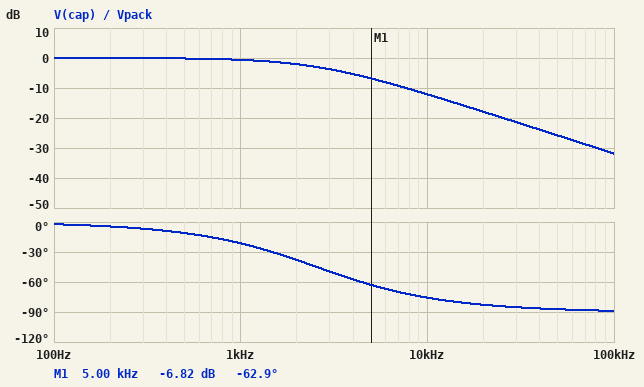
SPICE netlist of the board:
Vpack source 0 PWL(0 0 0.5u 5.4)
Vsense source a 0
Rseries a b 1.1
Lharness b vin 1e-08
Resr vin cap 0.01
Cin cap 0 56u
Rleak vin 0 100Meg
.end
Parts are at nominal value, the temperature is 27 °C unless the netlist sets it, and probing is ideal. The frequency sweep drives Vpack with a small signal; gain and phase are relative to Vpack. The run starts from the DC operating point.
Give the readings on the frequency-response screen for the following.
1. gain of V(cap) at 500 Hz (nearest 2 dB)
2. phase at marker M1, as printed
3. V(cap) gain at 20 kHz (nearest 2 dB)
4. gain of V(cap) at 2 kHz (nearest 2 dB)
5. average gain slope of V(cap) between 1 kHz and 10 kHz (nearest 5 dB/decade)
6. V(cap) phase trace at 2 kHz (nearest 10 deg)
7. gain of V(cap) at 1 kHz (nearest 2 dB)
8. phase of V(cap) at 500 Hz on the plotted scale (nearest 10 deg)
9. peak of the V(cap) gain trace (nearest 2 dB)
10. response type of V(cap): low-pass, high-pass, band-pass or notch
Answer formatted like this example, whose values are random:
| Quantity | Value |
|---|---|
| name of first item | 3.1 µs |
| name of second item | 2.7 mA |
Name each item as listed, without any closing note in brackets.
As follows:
| Quantity | Value |
|---|---|
| gain of V(cap) at 500 Hz | 0 dB |
| phase at marker M1, as printed | -62.9 deg |
| V(cap) gain at 20 kHz | -18 dB |
| gain of V(cap) at 2 kHz | -2 dB |
| average gain slope of V(cap) between 1 kHz and 10 kHz | -10 dB/decade |
| V(cap) phase trace at 2 kHz | -40 deg |
| gain of V(cap) at 1 kHz | 0 dB |
| phase of V(cap) at 500 Hz on the plotted scale | -10 deg |
| peak of the V(cap) gain trace | 0 dB |
| response type of V(cap): low-pass, high-pass, band-pass or notch | low-pass |
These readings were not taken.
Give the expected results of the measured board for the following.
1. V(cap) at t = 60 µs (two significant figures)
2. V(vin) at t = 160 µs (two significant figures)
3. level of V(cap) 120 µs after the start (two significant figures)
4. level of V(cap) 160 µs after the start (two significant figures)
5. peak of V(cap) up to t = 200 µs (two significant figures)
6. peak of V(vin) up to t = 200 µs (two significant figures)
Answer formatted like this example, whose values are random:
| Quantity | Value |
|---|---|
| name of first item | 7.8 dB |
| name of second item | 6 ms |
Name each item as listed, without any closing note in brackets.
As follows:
| Quantity | Value |
|---|---|
| V(cap) at t = 60 µs | 3.3 V |
| V(vin) at t = 160 µs | 5.0 V |
| level of V(cap) 120 µs after the start | 4.6 V |
| level of V(cap) 160 µs after the start | 5.0 V |
| peak of V(cap) up to t = 200 µs | 5.2 V |
| peak of V(vin) up to t = 200 µs | 5.2 V |
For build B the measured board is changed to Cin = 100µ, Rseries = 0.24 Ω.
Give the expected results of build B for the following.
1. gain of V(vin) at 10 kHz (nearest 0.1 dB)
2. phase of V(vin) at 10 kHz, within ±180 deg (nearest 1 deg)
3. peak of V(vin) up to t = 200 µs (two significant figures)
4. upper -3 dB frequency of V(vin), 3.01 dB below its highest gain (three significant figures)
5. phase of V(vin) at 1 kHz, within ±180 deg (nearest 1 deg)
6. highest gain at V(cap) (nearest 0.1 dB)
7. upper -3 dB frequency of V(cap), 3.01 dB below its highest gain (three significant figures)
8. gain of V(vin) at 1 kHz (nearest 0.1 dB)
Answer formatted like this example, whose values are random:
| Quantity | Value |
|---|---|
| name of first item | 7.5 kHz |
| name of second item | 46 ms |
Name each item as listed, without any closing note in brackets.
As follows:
| Quantity | Value |
|---|---|
| gain of V(vin) at 10 kHz | -5.4 dB |
| phase of V(vin) at 10 kHz, within ±180 deg | -54 deg |
| peak of V(vin) up to t = 200 µs | 5.4 V |
| upper -3 dB frequency of V(vin), 3.01 dB below its highest gain | 6.39 kHz |
| phase of V(vin) at 1 kHz, within ±180 deg | -9 deg |
| highest gain at V(cap) | 0 dB |
| upper -3 dB frequency of V(cap), 3.01 dB below its highest gain | 6.38 kHz |
| gain of V(vin) at 1 kHz | -0.1 dB |
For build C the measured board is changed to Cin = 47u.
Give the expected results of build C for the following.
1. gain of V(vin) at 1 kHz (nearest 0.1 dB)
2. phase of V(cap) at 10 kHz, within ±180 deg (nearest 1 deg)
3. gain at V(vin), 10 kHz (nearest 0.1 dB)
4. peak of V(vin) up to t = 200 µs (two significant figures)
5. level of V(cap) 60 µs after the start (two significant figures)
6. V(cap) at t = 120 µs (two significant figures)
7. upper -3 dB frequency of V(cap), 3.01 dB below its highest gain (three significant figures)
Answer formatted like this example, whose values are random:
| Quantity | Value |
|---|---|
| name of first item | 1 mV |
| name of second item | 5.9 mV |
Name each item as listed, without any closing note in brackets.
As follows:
| Quantity | Value |
|---|---|
| gain of V(vin) at 1 kHz | -0.4 dB |
| phase of V(cap) at 10 kHz, within ±180 deg | -73 deg |
| gain at V(vin), 10 kHz | -10.7 dB |
| peak of V(vin) up to t = 200 µs | 5.3 V |
| level of V(cap) 60 µs after the start | 3.7 V |
| V(cap) at t = 120 µs | 4.9 V |
| upper -3 dB frequency of V(cap), 3.01 dB below its highest gain | 3.05 kHz |
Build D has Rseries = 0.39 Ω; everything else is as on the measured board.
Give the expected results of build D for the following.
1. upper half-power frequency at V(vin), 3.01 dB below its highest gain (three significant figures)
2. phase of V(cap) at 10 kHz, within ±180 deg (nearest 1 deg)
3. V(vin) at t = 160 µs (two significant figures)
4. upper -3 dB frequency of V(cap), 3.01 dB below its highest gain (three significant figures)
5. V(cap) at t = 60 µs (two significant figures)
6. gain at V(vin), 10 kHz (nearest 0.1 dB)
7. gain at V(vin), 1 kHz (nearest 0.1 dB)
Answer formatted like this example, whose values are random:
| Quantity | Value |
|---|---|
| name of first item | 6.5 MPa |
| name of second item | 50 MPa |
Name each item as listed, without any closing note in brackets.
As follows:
| Quantity | Value |
|---|---|
| upper half-power frequency at V(vin), 3.01 dB below its highest gain | 7.12 kHz |
| phase of V(cap) at 10 kHz, within ±180 deg | -55 deg |
| V(vin) at t = 160 µs | 5.4 V |
| upper -3 dB frequency of V(cap), 3.01 dB below its highest gain | 7.11 kHz |
| V(cap) at t = 60 µs | 5.0 V |
| gain at V(vin), 10 kHz | -4.7 dB |
| gain at V(vin), 1 kHz | -0.1 dB |
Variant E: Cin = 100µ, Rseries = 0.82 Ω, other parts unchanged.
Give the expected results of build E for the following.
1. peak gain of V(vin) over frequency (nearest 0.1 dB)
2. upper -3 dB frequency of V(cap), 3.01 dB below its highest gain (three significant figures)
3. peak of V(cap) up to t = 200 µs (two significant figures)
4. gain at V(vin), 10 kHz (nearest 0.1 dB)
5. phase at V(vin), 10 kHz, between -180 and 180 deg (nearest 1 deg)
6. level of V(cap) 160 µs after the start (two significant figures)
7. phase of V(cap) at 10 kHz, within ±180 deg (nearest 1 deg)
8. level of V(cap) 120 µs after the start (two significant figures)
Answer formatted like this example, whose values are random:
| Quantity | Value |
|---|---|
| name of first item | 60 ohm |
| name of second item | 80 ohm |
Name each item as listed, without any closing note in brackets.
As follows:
| Quantity | Value |
|---|---|
| peak gain of V(vin) over frequency | 0 dB |
| upper -3 dB frequency of V(cap), 3.01 dB below its highest gain | 1.92 kHz |
| peak of V(cap) up to t = 200 µs | 4.9 V |
| gain at V(vin), 10 kHz | -14.5 dB |
| phase at V(vin), 10 kHz, between -180 and 180 deg | -76 deg |
| level of V(cap) 160 µs after the start | 4.6 V |
| phase of V(cap) at 10 kHz, within ±180 deg | -79 deg |
| level of V(cap) 120 µs after the start | 4.1 V |
